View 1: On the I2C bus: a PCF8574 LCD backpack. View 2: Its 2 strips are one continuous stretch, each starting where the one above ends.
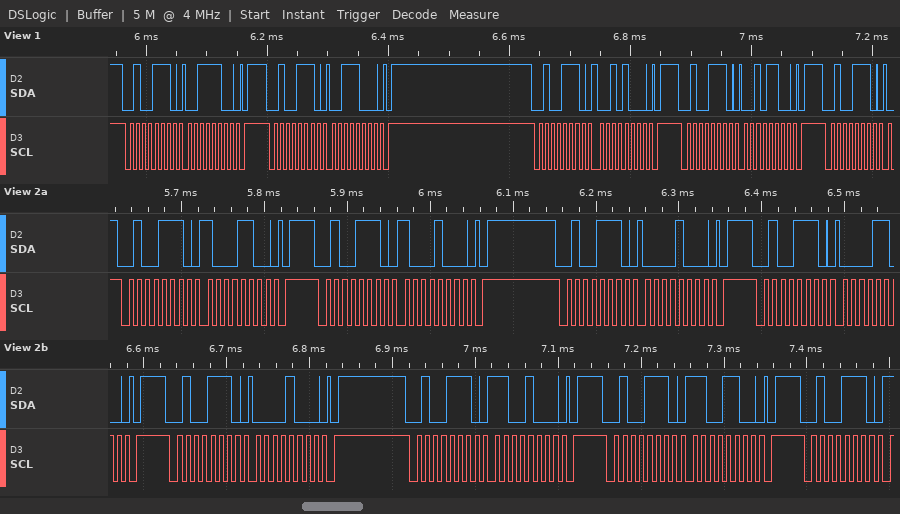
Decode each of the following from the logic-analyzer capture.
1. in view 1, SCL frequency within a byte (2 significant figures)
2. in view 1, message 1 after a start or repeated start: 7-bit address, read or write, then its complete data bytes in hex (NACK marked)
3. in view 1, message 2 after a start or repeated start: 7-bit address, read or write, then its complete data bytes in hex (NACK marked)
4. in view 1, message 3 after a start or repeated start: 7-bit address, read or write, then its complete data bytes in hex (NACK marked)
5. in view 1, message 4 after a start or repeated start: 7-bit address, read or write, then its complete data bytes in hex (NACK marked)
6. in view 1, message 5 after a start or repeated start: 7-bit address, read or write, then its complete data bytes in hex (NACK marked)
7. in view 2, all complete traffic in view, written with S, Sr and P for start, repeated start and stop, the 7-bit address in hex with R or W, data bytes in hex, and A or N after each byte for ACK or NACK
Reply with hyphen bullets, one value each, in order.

- 100 kHz
- 0x27 write: 3C
- 0x27 write: 38
- 0x27 write: 28
- 0x27 write: 2C
- 0x27 write
- S 27W A 8C A P S 27W A 88 A P S 27W A 08 A P S 27W A 0C A P S 27W A 08 A P S 27W A C8 A P S 27W A CC A P S 27W A
